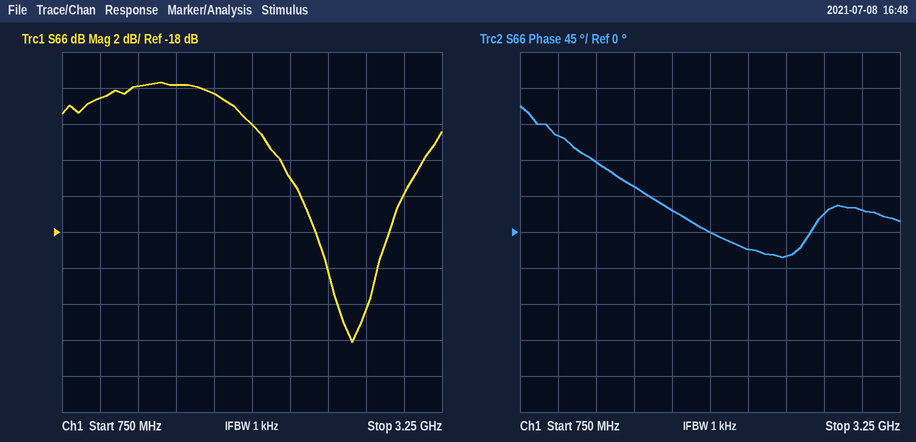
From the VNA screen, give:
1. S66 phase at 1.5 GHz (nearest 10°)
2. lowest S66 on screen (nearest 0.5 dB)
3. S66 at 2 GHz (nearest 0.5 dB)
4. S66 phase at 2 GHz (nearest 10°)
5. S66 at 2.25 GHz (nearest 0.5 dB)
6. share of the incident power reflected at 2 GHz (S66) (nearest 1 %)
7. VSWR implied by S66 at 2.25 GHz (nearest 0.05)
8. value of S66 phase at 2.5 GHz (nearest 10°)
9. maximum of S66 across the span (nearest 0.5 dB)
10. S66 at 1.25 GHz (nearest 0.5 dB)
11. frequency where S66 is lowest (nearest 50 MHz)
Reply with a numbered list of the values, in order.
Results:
1. 60°
2. -24.0 dB
3. -12.0 dB
4. 0°
5. -15.0 dB
6. 6 %
7. 1.45
8. -30°
9. -9.5 dB
10. -10.0 dB
11. 2.65 GHz
